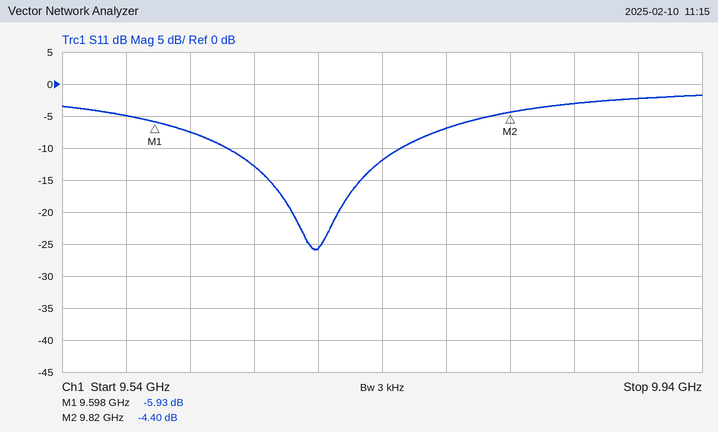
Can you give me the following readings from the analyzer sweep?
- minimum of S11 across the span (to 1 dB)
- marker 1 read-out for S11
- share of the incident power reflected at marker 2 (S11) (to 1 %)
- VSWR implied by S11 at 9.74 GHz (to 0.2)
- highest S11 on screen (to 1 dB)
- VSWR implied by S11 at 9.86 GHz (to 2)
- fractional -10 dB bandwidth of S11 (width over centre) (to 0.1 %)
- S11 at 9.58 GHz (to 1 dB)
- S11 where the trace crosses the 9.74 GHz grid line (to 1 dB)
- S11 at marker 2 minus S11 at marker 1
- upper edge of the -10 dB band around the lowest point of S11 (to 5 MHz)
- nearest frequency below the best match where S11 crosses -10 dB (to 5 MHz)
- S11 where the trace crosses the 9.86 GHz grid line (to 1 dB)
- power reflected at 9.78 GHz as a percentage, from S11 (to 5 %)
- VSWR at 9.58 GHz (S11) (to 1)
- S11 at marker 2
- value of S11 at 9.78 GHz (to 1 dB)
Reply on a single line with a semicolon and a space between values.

-26 dB; -5.93 dB; 36 %; 1.6; -2 dB; 6; 1.1 %; -5 dB; -12 dB; 1.53 dB; 9.750 GHz; 9.645 GHz; -3 dB; 20 %; 4; -4.40 dB; -7 dB
